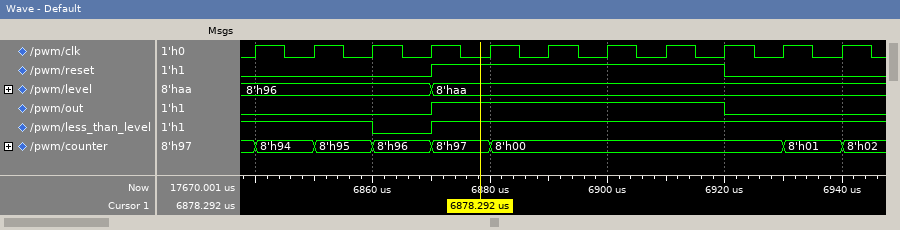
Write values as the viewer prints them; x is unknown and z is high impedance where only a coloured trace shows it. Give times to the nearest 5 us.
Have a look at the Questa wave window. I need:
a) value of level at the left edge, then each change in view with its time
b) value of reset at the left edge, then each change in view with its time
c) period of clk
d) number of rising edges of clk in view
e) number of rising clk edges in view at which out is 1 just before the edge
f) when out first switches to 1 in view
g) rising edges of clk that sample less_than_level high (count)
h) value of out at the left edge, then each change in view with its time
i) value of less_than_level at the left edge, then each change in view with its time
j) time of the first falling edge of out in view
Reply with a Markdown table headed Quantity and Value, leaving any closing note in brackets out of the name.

| Quantity | Value |
|---|---|
| value of level at the left edge, then each change in view with its time | 8'h96, 8'haa at 6870 us |
| value of reset at the left edge, then each change in view with its time | 0, 1 at 6870 us, 0 at 6920 us |
| period of clk | 10 us |
| number of rising edges of clk in view | 11 |
| number of rising clk edges in view at which out is 1 just before the edge | 5 |
| when out first switches to 1 in view | 6870 us |
| rising edges of clk that sample less_than_level high | 10 |
| value of out at the left edge, then each change in view with its time | 0, 1 at 6870 us, 0 at 6920 us |
| value of less_than_level at the left edge, then each change in view with its time | 1, 0 at 6860 us, 1 at 6870 us |
| time of the first falling edge of out in view | 6920 us |
